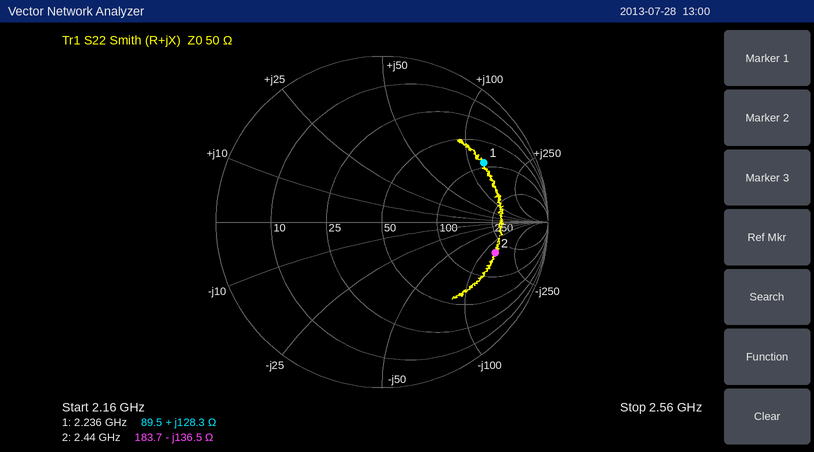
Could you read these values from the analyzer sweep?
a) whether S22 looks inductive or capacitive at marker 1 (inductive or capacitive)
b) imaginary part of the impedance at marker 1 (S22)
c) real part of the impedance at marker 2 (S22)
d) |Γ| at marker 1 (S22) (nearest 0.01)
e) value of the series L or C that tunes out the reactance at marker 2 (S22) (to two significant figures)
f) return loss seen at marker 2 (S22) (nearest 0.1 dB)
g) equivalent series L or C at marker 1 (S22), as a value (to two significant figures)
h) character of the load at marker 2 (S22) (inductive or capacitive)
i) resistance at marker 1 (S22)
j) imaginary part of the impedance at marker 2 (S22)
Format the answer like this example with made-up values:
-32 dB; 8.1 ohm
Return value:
inductive; +128.3 Ω; 183.7 Ω; 0.71; 8.9 nH; 3.0 dB; 9.1 nH; capacitive; 89.5 Ω; -136.5 Ω
